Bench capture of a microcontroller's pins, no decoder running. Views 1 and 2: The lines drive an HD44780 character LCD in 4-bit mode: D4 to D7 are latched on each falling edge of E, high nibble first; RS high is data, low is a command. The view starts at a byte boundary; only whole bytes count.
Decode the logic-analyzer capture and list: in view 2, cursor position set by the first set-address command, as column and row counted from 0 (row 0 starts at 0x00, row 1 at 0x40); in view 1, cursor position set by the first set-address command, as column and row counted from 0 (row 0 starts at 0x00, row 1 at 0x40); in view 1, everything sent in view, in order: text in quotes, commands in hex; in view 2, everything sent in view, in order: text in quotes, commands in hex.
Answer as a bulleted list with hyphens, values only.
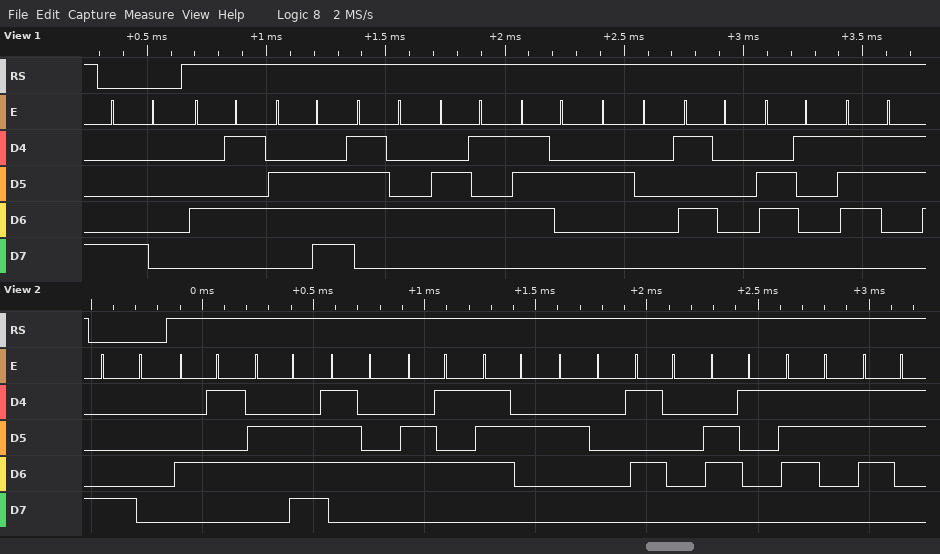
- column 0, row 0
- column 0, row 0
- 0x80 "Enter Pas"
- 0x80 "Enter Pass"
